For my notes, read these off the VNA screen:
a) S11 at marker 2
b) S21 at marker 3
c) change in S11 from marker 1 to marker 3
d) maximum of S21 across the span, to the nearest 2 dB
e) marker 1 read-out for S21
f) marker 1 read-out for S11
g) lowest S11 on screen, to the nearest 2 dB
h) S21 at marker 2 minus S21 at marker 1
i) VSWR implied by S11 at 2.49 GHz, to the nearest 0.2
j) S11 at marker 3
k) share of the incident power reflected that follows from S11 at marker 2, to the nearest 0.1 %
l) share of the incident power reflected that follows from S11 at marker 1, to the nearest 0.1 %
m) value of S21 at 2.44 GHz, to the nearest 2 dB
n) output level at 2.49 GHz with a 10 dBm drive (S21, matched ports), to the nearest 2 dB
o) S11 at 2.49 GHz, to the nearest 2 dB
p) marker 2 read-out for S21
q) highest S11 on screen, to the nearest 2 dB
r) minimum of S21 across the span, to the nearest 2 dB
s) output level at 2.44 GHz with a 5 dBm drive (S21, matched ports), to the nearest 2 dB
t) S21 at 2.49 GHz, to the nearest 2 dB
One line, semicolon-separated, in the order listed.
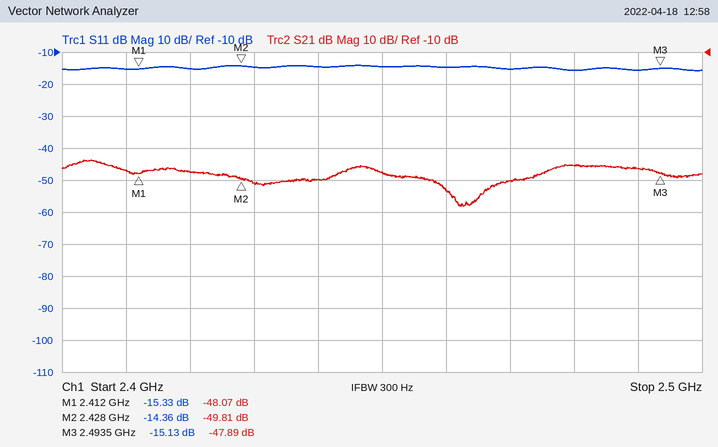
-14.36 dB; -47.89 dB; 0.20 dB; -44 dB; -48.07 dB; -15.33 dB; -16 dB; -1.74 dB; 1.4; -15.13 dB; 3.7 %; 2.9 %; -50 dB; -36 dBm; -16 dB; -49.81 dB; -14 dB; -58 dB; -44 dBm; -46 dB
